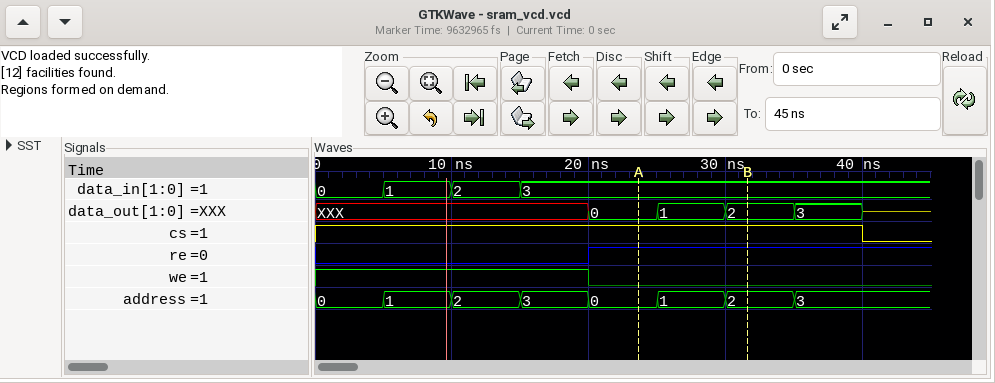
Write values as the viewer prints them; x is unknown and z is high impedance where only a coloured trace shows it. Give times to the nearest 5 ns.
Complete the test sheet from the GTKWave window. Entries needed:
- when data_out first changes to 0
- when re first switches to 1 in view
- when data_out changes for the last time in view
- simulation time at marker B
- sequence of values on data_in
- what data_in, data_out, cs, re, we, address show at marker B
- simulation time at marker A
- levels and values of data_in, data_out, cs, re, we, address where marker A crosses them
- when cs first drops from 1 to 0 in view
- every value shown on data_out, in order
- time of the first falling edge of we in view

20 ns
20 ns
40 ns
30 ns
0, 1, 2, 3
data_in=3, data_out=2, cs=1, re=1, we=0, address=2
25 ns
data_in=3, data_out=0, cs=1, re=1, we=0, address=0
40 ns
XXX, 0, 1, 2, 3, z
20 ns
